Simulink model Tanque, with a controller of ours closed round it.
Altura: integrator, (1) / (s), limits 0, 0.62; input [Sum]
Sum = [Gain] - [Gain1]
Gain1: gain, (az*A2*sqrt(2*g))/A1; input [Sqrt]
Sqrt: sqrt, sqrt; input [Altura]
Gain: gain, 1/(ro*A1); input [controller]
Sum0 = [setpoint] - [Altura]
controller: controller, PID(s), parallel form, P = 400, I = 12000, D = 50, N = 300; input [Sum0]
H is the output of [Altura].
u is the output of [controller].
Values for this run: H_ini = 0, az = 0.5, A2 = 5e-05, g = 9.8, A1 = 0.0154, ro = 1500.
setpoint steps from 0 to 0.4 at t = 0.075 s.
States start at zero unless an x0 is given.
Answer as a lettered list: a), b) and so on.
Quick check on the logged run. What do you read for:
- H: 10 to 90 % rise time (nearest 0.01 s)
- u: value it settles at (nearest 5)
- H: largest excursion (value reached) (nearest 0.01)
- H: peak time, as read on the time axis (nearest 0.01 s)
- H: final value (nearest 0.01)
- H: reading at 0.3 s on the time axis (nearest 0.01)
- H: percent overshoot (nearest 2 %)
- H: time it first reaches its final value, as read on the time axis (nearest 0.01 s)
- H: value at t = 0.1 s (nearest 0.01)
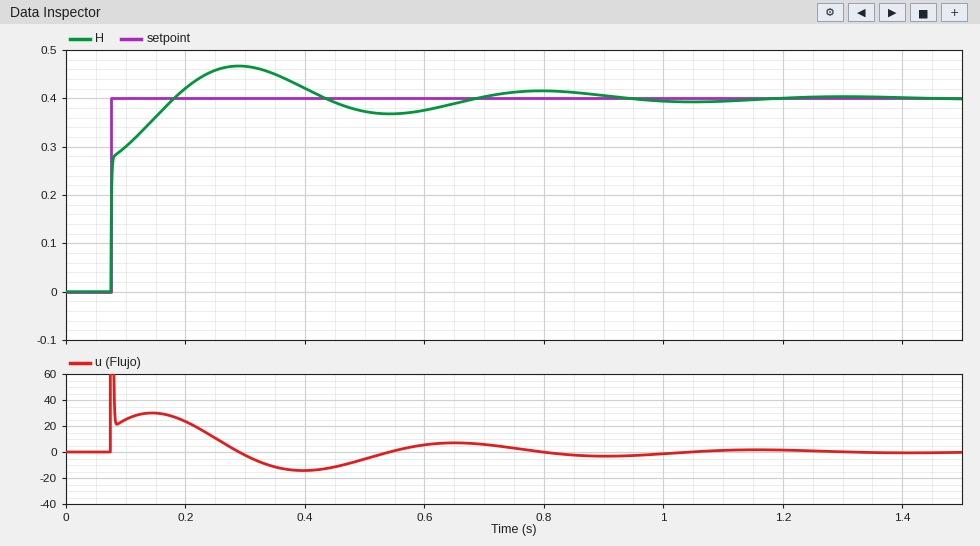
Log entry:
a) 0.07 s
b) 0
c) 0.47
d) 0.29 s
e) 0.40
f) 0.47
g) 16 %
h) 0.18 s
i) 0.30
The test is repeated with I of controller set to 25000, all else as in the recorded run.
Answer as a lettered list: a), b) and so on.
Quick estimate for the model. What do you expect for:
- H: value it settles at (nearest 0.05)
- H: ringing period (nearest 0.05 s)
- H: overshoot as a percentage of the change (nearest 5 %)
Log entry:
a) 0.40
b) 0.35 s
c) 20 %
